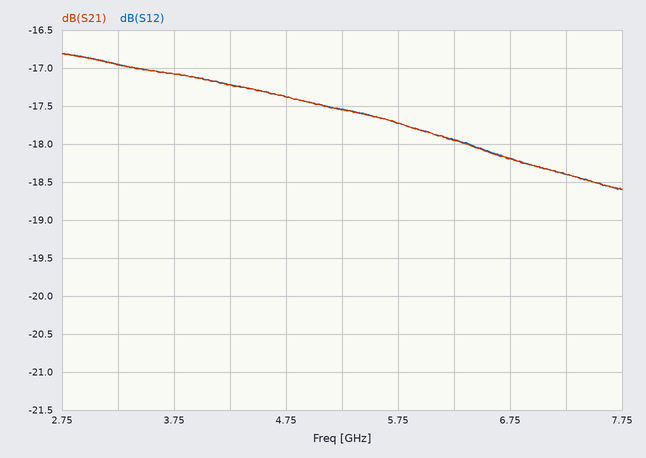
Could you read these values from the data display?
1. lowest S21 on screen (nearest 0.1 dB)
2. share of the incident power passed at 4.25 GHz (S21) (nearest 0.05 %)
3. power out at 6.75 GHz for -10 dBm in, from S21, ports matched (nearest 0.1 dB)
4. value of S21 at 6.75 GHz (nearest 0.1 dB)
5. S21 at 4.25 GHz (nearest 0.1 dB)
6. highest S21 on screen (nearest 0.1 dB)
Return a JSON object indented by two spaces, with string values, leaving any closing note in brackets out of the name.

{
  "lowest S21 on screen": "-18.6 dB",
  "share of the incident power passed at 4.25 GHz (S21)": "1.90 %",
  "power out at 6.75 GHz for -10 dBm in, from S21, ports matched": "-28.2 dBm",
  "value of S21 at 6.75 GHz": "-18.2 dB",
  "S21 at 4.25 GHz": "-17.2 dB",
  "highest S21 on screen": "-16.8 dB"
}
